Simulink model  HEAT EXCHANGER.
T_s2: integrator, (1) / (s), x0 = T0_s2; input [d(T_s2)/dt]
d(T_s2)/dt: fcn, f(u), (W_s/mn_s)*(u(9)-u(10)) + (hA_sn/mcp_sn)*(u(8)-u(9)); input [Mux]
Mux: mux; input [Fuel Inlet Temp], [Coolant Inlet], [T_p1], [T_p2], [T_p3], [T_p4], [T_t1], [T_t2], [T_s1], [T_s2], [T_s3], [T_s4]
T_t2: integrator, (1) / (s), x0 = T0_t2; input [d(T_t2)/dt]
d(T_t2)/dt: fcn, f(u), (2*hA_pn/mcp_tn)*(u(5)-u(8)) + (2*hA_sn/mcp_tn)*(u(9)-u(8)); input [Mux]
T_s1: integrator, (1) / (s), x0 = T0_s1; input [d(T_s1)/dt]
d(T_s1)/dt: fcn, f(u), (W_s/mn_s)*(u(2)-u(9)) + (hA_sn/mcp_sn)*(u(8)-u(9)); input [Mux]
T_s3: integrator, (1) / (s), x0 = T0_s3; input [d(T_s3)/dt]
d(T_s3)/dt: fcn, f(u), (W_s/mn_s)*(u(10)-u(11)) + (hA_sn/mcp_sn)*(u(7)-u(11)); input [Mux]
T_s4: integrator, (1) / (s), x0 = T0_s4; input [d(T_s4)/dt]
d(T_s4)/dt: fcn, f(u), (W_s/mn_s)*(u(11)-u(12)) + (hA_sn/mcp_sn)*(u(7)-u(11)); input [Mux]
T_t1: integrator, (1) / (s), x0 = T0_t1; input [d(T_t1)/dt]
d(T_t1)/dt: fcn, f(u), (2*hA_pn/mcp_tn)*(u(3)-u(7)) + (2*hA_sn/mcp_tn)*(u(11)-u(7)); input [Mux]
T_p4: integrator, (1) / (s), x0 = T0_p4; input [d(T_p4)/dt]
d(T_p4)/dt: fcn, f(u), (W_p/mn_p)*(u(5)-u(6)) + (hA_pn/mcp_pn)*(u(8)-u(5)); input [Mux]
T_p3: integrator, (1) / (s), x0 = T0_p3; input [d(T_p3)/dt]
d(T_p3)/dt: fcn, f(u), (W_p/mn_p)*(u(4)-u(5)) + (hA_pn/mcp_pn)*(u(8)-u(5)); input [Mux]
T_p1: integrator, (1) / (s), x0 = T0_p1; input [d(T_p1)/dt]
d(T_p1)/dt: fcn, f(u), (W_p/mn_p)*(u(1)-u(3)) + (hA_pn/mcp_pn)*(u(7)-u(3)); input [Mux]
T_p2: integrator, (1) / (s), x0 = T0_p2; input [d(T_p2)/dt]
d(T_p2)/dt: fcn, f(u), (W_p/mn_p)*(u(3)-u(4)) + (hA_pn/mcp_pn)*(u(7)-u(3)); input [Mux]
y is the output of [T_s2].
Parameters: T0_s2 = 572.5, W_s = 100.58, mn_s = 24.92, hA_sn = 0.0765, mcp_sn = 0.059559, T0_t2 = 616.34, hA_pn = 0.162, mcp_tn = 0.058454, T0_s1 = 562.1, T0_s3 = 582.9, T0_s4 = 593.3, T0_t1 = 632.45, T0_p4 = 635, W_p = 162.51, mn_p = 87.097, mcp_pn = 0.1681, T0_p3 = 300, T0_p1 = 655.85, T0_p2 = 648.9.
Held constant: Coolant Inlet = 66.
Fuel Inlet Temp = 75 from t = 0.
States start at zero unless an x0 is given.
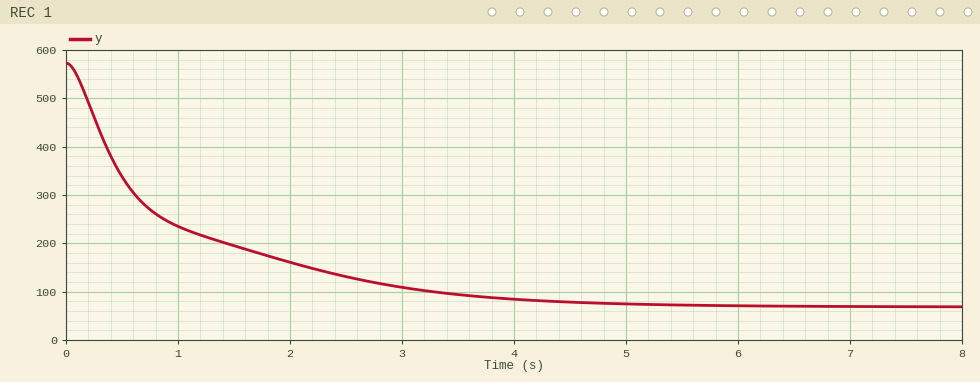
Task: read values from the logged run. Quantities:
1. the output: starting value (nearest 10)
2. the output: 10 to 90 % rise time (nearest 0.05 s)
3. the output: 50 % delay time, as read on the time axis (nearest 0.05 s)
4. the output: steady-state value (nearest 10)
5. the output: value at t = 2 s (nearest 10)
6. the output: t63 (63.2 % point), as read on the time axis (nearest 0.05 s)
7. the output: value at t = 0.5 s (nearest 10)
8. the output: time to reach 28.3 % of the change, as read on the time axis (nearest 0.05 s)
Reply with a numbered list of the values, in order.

1. 570
2. 2.60 s
3. 0.55 s
4. 70
5. 160
6. 0.85 s
7. 340
8. 0.30 s
